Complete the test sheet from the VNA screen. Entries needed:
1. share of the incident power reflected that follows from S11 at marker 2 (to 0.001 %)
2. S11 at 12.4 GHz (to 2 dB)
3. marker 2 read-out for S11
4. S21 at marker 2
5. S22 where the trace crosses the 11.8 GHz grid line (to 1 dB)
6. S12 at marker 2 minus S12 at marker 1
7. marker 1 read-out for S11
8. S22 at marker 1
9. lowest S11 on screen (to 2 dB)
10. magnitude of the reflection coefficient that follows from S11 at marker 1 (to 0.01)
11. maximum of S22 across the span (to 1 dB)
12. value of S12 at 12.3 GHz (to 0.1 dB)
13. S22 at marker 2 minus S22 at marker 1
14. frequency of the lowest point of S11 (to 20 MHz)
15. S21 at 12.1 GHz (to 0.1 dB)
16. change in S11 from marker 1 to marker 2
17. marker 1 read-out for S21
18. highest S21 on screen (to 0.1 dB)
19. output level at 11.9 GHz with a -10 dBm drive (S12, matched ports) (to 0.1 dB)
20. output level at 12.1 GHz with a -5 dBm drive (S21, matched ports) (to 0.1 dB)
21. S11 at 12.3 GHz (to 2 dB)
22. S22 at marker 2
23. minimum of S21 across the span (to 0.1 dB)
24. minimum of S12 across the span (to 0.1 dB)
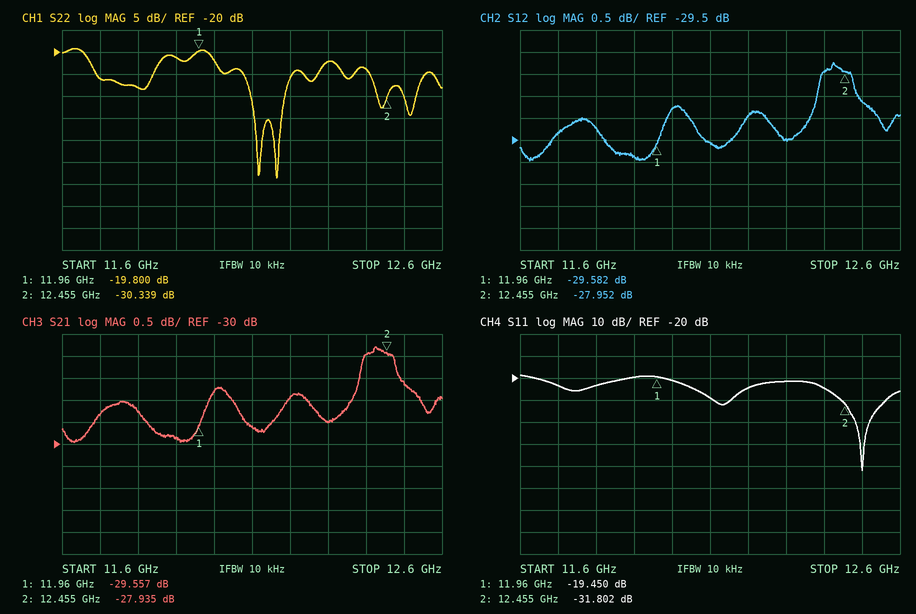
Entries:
0.066 %
-24 dB
-31.802 dB
-27.935 dB
-28 dB
1.630 dB
-19.450 dB
-19.800 dB
-62 dB
0.11
-19 dB
-29.5 dB
-10.539 dB
12.50 GHz
-29.6 dB
-12.352 dB
-29.557 dB
-27.8 dB
-39.9 dBm
-34.6 dBm
-22 dB
-30.339 dB
-30.0 dB
-30.0 dB
